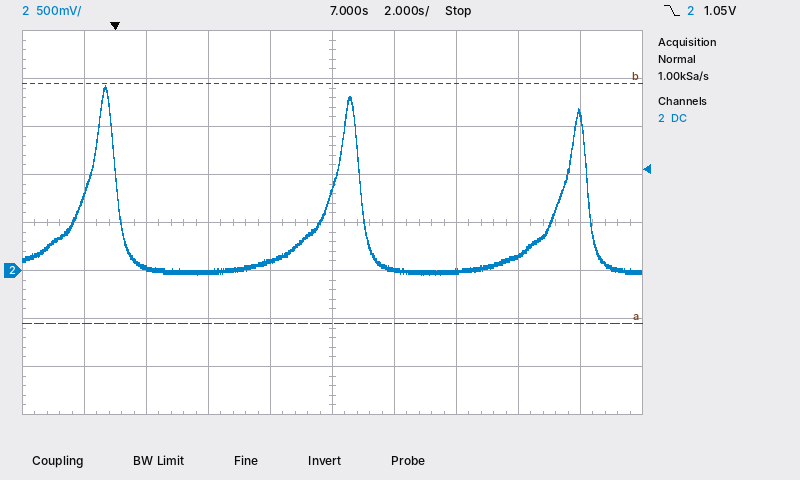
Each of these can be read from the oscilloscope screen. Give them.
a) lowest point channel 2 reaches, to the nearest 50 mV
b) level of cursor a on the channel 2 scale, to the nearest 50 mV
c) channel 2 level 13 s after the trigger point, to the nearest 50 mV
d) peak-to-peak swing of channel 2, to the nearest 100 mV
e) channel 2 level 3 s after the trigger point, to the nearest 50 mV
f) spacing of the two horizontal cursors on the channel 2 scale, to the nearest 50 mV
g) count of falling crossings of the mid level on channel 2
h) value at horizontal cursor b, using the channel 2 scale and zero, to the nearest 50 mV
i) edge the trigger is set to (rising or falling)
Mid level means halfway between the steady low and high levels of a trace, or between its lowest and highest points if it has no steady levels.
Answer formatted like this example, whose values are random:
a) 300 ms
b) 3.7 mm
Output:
a) -50 mV
b) -550 mV
c) 150 mV
d) 2.00 V
e) 0 mV
f) 2.50 V
g) 3
h) 1.95 V
i) falling
